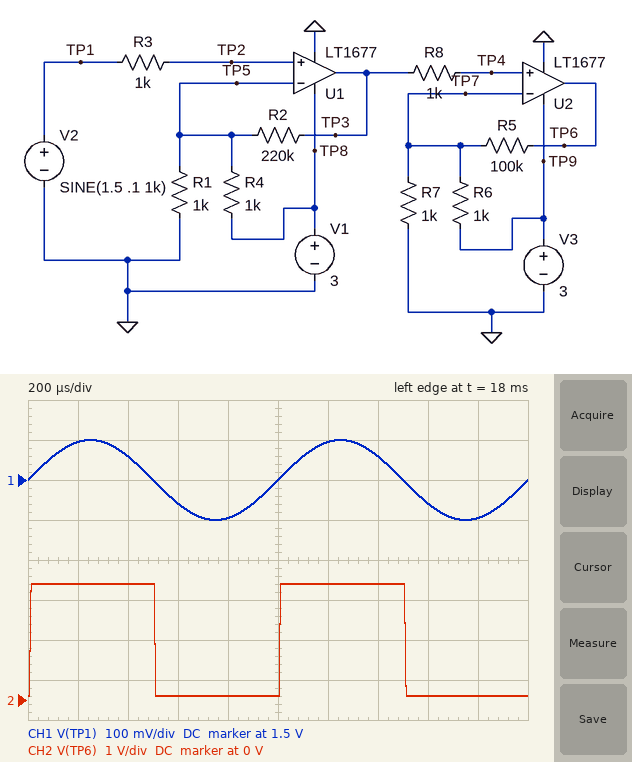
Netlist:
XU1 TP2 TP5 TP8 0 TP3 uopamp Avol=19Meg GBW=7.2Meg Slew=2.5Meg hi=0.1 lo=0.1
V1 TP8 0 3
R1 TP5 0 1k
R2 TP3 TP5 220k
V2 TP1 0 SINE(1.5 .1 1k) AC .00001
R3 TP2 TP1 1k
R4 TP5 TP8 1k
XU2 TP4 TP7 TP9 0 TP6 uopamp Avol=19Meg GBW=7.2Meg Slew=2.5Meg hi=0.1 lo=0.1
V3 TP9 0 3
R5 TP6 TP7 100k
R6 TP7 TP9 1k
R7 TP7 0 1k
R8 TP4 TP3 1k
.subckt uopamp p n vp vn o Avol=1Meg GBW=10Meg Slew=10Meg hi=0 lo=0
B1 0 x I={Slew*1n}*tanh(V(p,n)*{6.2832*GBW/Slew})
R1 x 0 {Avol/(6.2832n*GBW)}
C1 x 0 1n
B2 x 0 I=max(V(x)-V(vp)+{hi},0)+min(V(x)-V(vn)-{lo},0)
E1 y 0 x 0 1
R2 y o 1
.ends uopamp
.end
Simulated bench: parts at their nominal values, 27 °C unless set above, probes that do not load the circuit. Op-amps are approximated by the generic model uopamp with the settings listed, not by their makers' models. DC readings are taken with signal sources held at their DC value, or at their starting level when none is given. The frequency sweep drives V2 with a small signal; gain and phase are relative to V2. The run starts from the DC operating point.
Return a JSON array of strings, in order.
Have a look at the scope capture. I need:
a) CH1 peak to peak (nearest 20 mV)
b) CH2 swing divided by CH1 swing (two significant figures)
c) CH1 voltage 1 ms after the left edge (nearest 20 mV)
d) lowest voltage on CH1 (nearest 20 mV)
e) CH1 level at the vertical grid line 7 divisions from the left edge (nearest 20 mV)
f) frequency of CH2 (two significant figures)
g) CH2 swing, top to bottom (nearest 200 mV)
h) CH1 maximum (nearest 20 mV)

["200 mV", "14", "1.50 V", "1.40 V", "1.56 V", "1.0 kHz", "2.8 V", "1.60 V"]
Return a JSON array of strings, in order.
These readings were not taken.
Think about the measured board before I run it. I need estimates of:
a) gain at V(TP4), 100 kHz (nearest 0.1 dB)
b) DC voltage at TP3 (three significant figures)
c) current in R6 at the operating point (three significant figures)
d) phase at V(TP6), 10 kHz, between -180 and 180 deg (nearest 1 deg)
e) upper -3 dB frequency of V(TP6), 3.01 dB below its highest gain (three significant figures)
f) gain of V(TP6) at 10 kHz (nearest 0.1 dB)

["37.0 dB", "1.50 V", "1.50 mA", "-47 deg", "14.0 kHz", "97.2 dB"]
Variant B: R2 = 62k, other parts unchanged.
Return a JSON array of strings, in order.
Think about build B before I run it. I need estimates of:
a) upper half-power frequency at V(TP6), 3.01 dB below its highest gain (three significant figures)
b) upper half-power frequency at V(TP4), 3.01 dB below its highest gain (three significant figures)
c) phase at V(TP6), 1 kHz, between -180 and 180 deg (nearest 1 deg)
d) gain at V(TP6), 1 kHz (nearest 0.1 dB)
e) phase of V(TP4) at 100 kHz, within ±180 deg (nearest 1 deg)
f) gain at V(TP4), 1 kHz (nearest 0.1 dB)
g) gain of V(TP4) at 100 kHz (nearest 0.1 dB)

["28.1 kHz", "57.6 kHz", "-3 deg", "88.0 dB", "-60 deg", "41.9 dB", "35.9 dB"]
